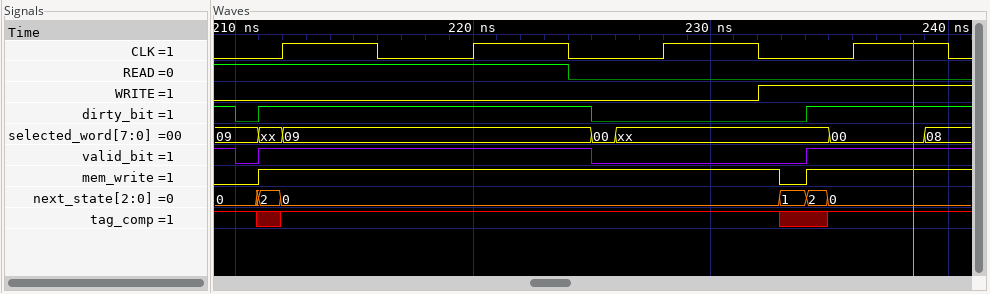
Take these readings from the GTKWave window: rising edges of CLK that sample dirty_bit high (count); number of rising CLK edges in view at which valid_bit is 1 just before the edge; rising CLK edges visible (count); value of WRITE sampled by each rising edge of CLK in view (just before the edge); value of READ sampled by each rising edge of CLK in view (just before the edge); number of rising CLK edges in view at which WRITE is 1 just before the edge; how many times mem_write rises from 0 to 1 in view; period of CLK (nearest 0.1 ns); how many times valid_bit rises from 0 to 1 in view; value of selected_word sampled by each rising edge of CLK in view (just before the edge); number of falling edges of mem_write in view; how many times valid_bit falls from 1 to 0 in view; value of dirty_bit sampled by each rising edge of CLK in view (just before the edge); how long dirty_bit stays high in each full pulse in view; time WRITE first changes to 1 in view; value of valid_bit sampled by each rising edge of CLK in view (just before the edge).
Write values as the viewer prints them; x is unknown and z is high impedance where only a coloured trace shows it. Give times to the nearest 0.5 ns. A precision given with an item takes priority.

3
3
4
0 0 0 1
1 1 0 0
1
2
8 ns
2
xx, 09, xx, 00
1
2
1 1 0 1
14 ns
232 ns
1 1 0 1
